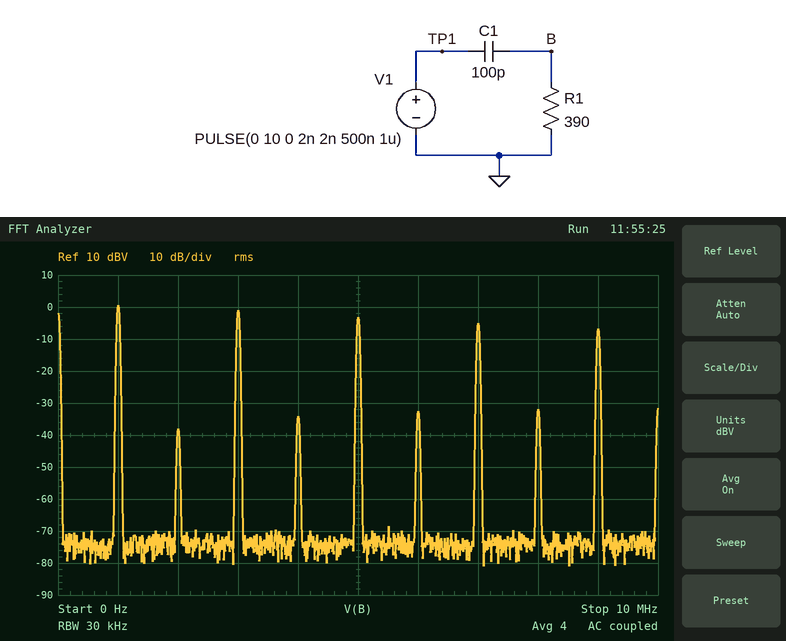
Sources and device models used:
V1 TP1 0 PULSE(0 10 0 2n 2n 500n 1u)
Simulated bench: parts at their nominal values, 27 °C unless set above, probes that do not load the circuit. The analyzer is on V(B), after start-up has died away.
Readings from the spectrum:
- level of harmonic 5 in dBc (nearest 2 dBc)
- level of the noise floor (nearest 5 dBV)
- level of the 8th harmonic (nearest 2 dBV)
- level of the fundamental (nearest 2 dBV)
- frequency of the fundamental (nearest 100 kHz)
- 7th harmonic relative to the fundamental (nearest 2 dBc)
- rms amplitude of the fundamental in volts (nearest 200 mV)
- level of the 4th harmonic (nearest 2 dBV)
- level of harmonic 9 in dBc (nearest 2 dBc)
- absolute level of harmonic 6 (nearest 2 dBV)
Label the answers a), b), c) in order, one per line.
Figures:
a) -4 dBc
b) -75 dBV
c) -32 dBV
d) 0 dBV
e) 1.0 MHz
f) -6 dBc
g) 1.0 V
h) -34 dBV
i) -8 dBc
j) -32 dBV
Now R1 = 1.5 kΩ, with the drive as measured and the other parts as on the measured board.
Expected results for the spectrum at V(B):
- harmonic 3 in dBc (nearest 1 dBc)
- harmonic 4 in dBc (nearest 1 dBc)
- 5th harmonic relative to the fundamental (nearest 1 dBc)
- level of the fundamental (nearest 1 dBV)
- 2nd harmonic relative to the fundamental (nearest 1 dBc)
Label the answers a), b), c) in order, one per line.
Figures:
a) -7 dBc
b) -41 dBc
c) -11 dBc
d) 10 dBV
e) -42 dBc
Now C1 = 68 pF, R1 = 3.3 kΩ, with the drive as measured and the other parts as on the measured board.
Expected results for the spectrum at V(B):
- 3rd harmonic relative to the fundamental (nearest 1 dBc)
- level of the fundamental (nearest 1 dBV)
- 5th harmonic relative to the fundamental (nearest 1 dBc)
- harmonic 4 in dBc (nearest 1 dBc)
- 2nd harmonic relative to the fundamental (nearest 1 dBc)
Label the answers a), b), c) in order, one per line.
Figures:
a) -8 dBc
b) 11 dBV
c) -12 dBc
d) -42 dBc
e) -43 dBc
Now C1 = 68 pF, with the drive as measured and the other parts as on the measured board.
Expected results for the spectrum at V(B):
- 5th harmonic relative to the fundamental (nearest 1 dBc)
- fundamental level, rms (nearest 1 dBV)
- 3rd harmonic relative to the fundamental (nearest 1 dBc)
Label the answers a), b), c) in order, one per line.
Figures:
a) -2 dBc
b) -3 dBV
c) -1 dBc
